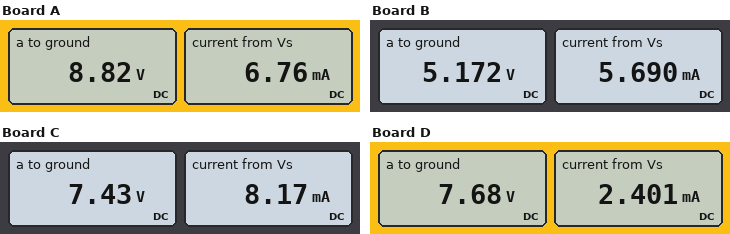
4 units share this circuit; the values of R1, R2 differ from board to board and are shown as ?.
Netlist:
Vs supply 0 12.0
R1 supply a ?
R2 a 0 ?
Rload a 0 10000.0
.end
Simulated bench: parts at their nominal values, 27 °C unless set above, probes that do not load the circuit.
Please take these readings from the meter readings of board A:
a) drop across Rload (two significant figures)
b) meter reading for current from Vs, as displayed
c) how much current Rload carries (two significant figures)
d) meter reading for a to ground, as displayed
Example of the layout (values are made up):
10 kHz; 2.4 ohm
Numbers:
8.8 V; 6.76 mA; 880 µA; 8.82 V
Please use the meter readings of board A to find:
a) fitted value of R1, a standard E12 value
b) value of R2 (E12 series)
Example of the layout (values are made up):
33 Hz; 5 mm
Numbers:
470 Ω; 1.5 kΩ
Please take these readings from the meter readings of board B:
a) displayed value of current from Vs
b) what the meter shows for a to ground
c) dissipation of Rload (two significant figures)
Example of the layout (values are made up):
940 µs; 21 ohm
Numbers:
5.690 mA; 5.172 V; 2.7 mW
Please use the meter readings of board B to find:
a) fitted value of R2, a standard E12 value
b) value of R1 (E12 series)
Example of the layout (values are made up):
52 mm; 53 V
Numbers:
1 kΩ; 1.2 kΩ
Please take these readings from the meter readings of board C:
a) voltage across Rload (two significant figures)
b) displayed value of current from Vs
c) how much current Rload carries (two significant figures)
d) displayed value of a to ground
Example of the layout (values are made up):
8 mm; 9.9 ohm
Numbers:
7.4 V; 8.17 mA; 740 µA; 7.43 V
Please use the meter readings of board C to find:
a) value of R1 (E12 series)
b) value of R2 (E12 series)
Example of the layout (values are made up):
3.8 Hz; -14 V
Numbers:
560 Ω; 1 kΩ
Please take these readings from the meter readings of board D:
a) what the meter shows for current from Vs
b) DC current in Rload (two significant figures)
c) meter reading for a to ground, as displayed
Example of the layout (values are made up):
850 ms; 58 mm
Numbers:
2.401 mA; 770 µA; 7.68 V
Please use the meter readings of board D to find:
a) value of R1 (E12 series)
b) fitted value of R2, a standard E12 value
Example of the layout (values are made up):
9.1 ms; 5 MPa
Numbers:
1.8 kΩ; 4.7 kΩ
